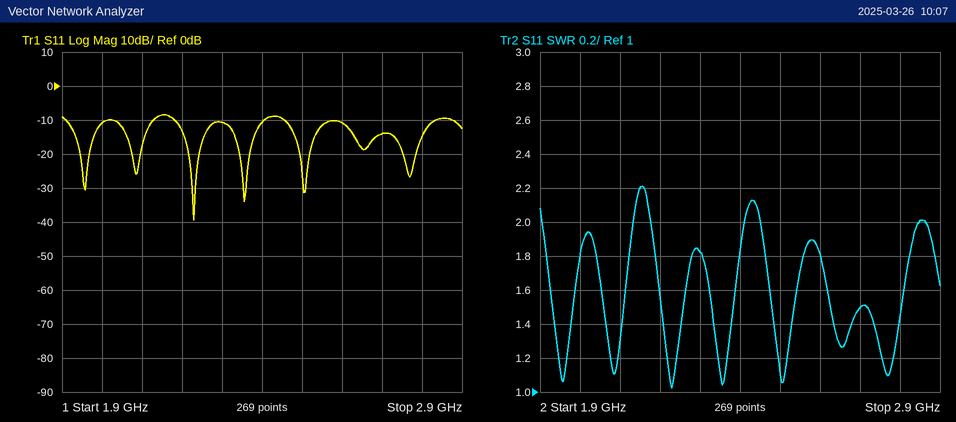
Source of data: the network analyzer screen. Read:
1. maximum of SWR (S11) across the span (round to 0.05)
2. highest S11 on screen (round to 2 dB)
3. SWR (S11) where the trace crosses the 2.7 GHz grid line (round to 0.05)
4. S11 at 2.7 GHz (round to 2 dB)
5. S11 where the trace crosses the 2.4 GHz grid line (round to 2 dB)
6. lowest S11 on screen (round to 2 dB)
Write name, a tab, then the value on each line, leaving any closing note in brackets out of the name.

maximum of SWR (S11) across the span	2.20
highest S11 on screen	-8 dB
SWR (S11) where the trace crosses the 2.7 GHz grid line	1.50
S11 at 2.7 GHz	-14 dB
S11 where the trace crosses the 2.4 GHz grid line	-10 dB
lowest S11 on screen	-40 dB
